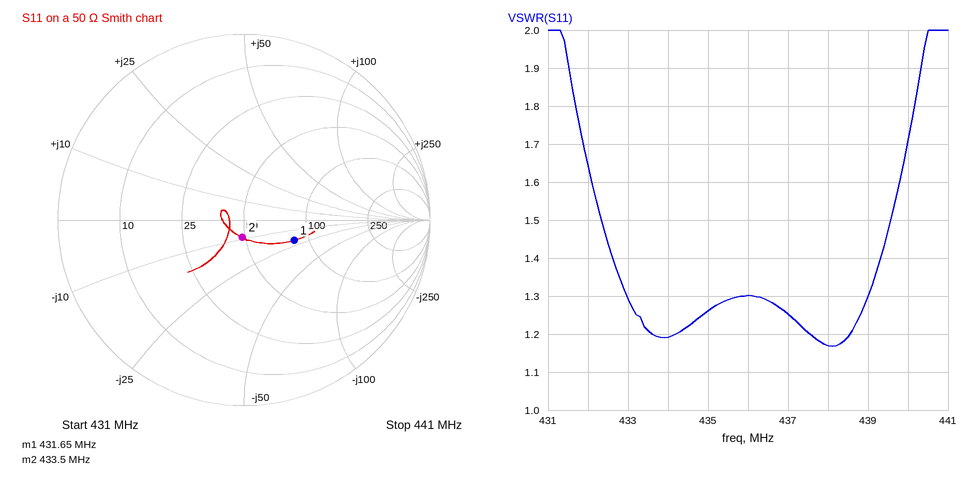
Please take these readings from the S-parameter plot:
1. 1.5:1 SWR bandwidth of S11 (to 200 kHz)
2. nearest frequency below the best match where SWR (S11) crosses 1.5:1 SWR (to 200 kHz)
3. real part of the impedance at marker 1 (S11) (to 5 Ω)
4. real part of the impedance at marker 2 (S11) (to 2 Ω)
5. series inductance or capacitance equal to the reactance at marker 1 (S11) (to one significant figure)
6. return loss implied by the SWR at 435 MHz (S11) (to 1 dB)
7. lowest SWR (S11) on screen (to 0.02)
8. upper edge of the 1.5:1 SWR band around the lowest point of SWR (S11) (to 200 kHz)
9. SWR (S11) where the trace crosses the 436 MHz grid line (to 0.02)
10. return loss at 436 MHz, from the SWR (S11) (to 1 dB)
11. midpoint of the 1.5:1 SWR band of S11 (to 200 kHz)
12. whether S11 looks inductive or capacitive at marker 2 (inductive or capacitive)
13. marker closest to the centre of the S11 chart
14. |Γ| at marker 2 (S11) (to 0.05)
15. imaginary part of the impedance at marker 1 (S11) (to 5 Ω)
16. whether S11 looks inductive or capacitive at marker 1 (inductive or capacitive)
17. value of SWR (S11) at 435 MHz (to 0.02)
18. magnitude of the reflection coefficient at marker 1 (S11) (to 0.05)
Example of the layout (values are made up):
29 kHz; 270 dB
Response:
7.2 MHz; 432.4 MHz; 85 Ω; 48 Ω; 20 pF; 19 dB; 1.16; 439.6 MHz; 1.30; 18 dB; 436.0 MHz; capacitive; marker 2; 0.10; -20 Ω; capacitive; 1.26; 0.30
